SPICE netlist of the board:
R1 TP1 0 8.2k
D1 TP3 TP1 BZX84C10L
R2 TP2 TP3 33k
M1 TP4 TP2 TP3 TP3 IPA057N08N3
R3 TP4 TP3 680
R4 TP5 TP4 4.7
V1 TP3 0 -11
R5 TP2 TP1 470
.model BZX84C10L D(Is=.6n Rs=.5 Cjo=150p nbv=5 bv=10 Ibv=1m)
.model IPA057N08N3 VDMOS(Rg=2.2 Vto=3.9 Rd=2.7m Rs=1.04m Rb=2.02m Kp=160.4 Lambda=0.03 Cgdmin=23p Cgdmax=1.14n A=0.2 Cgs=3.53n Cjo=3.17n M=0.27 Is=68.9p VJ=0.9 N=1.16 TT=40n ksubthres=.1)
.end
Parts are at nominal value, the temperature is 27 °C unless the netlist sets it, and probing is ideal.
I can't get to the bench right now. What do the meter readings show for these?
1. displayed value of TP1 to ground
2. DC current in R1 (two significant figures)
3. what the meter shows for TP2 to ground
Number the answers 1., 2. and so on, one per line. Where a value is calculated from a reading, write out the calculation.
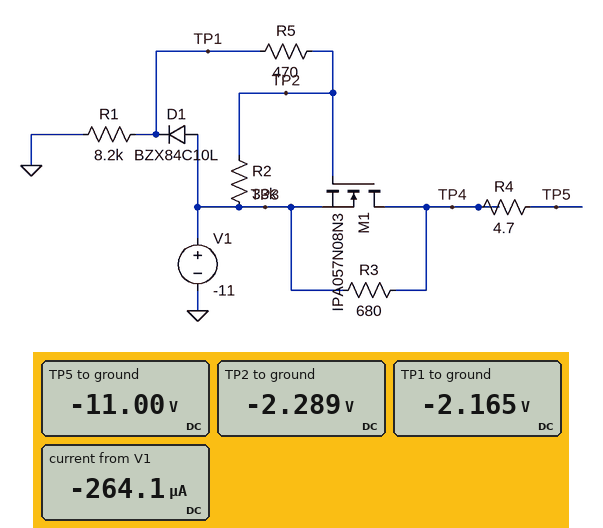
1. -2.165 V
2. (0 V - (-2.165 V)) / 8.2 kΩ = 260 µA
3. -2.289 V
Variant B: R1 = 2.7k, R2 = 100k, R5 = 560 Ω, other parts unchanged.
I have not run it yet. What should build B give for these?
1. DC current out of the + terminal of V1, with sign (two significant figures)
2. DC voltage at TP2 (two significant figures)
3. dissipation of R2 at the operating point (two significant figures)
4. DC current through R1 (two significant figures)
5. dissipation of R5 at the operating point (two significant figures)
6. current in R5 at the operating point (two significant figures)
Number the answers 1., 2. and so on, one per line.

1. -420 µA
2. -1.2 V
3. 960 µW
4. 420 µA
5. 5.4 µW
6. 98 µA
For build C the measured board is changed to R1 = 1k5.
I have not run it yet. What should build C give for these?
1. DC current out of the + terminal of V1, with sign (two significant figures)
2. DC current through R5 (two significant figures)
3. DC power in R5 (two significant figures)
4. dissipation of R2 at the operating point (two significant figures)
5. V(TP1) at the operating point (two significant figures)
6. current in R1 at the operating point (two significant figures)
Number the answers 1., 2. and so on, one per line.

1. -740 µA
2. 300 µA
3. 41 µW
4. 2.9 mW
5. -1.1 V
6. 740 µA
